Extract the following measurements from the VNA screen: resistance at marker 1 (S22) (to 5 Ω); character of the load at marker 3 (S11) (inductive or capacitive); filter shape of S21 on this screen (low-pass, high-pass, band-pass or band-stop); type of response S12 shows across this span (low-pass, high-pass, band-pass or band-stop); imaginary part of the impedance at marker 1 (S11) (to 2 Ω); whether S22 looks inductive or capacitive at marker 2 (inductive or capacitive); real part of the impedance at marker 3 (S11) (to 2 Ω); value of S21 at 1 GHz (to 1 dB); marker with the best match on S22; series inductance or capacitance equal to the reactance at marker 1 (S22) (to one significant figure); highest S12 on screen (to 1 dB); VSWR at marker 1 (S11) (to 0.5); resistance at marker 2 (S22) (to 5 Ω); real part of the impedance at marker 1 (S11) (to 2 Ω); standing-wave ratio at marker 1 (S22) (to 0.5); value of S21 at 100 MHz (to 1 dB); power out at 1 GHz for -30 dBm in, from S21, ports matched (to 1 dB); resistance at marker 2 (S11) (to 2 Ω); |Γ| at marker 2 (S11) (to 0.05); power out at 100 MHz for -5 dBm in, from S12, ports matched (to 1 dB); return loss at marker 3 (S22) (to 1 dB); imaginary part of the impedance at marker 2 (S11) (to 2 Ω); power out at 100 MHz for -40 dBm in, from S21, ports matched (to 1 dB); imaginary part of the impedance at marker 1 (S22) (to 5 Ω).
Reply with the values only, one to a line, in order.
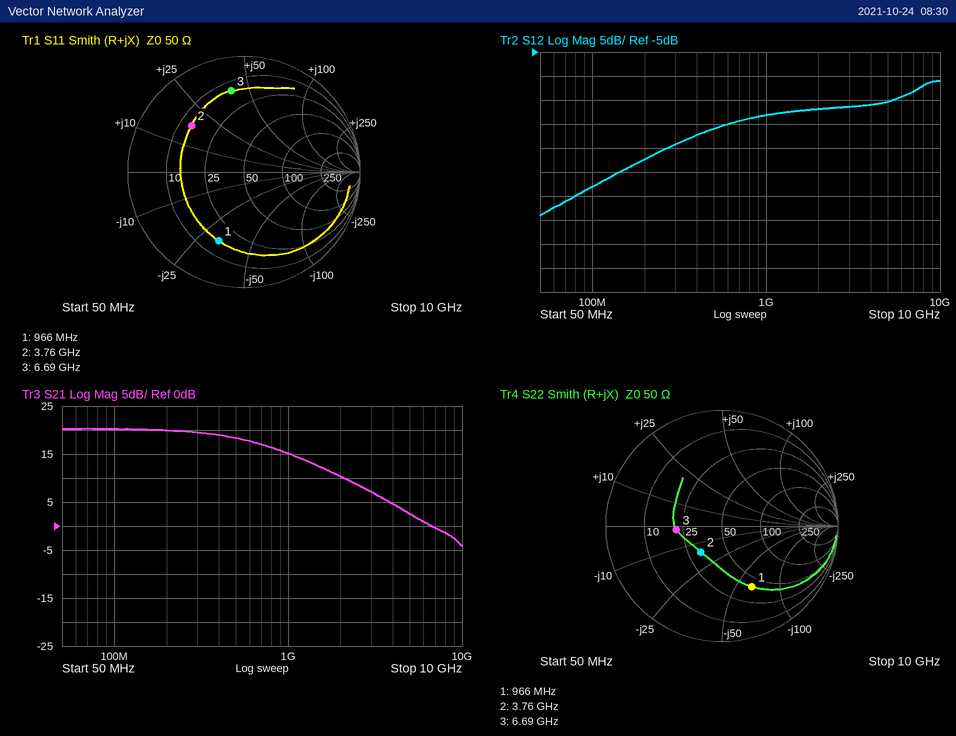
40 Ω
inductive
low-pass
high-pass
-32 Ω
capacitive
14 Ω
15 dB
marker 2
3 pF
-11 dB
4.5
30 Ω
16 Ω
4.0
20 dB
-15 dBm
14 Ω
0.60
-38 dBm
8 dB
+18 Ω
-20 dBm
-65 Ω
